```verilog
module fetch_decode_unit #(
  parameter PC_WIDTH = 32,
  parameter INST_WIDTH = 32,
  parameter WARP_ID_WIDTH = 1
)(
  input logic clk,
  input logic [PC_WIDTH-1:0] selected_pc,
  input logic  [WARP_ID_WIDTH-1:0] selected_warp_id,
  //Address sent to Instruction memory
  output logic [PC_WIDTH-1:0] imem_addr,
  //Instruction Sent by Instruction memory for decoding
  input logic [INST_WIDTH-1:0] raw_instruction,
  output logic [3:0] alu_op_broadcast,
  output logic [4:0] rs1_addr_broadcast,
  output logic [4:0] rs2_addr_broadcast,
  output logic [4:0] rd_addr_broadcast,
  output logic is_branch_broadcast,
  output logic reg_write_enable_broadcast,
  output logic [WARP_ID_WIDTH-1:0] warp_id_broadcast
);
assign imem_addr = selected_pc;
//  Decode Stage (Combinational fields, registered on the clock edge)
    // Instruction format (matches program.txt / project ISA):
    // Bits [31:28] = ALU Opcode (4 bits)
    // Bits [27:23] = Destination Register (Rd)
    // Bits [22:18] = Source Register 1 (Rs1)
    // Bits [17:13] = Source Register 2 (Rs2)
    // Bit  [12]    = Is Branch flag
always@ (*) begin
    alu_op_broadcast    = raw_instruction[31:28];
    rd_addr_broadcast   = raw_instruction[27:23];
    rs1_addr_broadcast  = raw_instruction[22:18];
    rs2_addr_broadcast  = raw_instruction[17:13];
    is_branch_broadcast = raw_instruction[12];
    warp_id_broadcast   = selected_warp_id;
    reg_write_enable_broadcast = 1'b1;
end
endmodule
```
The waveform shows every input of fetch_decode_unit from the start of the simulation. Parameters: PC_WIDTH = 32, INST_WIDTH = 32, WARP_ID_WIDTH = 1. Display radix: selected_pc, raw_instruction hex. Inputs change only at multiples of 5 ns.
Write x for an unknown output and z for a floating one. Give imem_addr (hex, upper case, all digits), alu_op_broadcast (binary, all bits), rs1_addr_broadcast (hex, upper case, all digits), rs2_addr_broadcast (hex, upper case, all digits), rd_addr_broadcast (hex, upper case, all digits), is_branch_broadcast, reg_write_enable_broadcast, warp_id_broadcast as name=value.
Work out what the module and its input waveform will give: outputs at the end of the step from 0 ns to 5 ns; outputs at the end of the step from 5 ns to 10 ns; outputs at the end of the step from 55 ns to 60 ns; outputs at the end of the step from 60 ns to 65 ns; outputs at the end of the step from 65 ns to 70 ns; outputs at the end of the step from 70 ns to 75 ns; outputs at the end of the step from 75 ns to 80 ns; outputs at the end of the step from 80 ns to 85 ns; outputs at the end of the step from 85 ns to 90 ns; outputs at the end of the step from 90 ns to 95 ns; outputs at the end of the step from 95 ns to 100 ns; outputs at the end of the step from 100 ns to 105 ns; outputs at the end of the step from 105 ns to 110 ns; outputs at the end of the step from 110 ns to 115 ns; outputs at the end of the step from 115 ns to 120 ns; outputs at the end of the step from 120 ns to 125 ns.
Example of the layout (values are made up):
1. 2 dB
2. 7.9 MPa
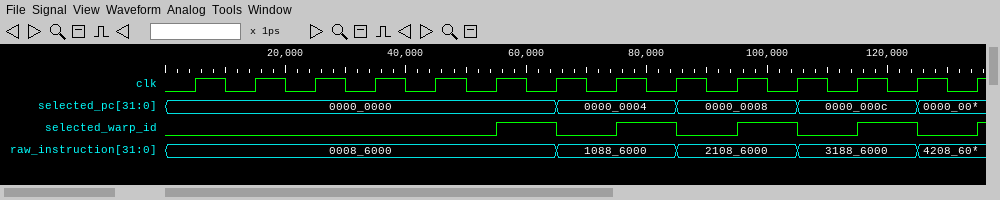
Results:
1. imem_addr=00000000, alu_op_broadcast=0000, rs1_addr_broadcast=02, rs2_addr_broadcast=03, rd_addr_broadcast=00, is_branch_broadcast=0, reg_write_enable_broadcast=1, warp_id_broadcast=0
2. imem_addr=00000000, alu_op_broadcast=0000, rs1_addr_broadcast=02, rs2_addr_broadcast=03, rd_addr_broadcast=00, is_branch_broadcast=0, reg_write_enable_broadcast=1, warp_id_broadcast=0
3. imem_addr=00000000, alu_op_broadcast=0000, rs1_addr_broadcast=02, rs2_addr_broadcast=03, rd_addr_broadcast=00, is_branch_broadcast=0, reg_write_enable_broadcast=1, warp_id_broadcast=1
4. imem_addr=00000000, alu_op_broadcast=0000, rs1_addr_broadcast=02, rs2_addr_broadcast=03, rd_addr_broadcast=00, is_branch_broadcast=0, reg_write_enable_broadcast=1, warp_id_broadcast=1
5. imem_addr=00000004, alu_op_broadcast=0001, rs1_addr_broadcast=02, rs2_addr_broadcast=03, rd_addr_broadcast=01, is_branch_broadcast=0, reg_write_enable_broadcast=1, warp_id_broadcast=0
6. imem_addr=00000004, alu_op_broadcast=0001, rs1_addr_broadcast=02, rs2_addr_broadcast=03, rd_addr_broadcast=01, is_branch_broadcast=0, reg_write_enable_broadcast=1, warp_id_broadcast=0
7. imem_addr=00000004, alu_op_broadcast=0001, rs1_addr_broadcast=02, rs2_addr_broadcast=03, rd_addr_broadcast=01, is_branch_broadcast=0, reg_write_enable_broadcast=1, warp_id_broadcast=1
8. imem_addr=00000004, alu_op_broadcast=0001, rs1_addr_broadcast=02, rs2_addr_broadcast=03, rd_addr_broadcast=01, is_branch_broadcast=0, reg_write_enable_broadcast=1, warp_id_broadcast=1
9. imem_addr=00000008, alu_op_broadcast=0010, rs1_addr_broadcast=02, rs2_addr_broadcast=03, rd_addr_broadcast=02, is_branch_broadcast=0, reg_write_enable_broadcast=1, warp_id_broadcast=0
10. imem_addr=00000008, alu_op_broadcast=0010, rs1_addr_broadcast=02, rs2_addr_broadcast=03, rd_addr_broadcast=02, is_branch_broadcast=0, reg_write_enable_broadcast=1, warp_id_broadcast=0
11. imem_addr=00000008, alu_op_broadcast=0010, rs1_addr_broadcast=02, rs2_addr_broadcast=03, rd_addr_broadcast=02, is_branch_broadcast=0, reg_write_enable_broadcast=1, warp_id_broadcast=1
12. imem_addr=00000008, alu_op_broadcast=0010, rs1_addr_broadcast=02, rs2_addr_broadcast=03, rd_addr_broadcast=02, is_branch_broadcast=0, reg_write_enable_broadcast=1, warp_id_broadcast=1
13. imem_addr=0000000C, alu_op_broadcast=0011, rs1_addr_broadcast=02, rs2_addr_broadcast=03, rd_addr_broadcast=03, is_branch_broadcast=0, reg_write_enable_broadcast=1, warp_id_broadcast=0
14. imem_addr=0000000C, alu_op_broadcast=0011, rs1_addr_broadcast=02, rs2_addr_broadcast=03, rd_addr_broadcast=03, is_branch_broadcast=0, reg_write_enable_broadcast=1, warp_id_broadcast=0
15. imem_addr=0000000C, alu_op_broadcast=0011, rs1_addr_broadcast=02, rs2_addr_broadcast=03, rd_addr_broadcast=03, is_branch_broadcast=0, reg_write_enable_broadcast=1, warp_id_broadcast=1
16. imem_addr=0000000C, alu_op_broadcast=0011, rs1_addr_broadcast=02, rs2_addr_broadcast=03, rd_addr_broadcast=03, is_branch_broadcast=0, reg_write_enable_broadcast=1, warp_id_broadcast=1
